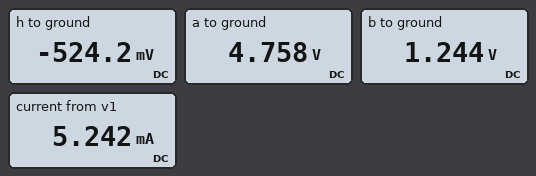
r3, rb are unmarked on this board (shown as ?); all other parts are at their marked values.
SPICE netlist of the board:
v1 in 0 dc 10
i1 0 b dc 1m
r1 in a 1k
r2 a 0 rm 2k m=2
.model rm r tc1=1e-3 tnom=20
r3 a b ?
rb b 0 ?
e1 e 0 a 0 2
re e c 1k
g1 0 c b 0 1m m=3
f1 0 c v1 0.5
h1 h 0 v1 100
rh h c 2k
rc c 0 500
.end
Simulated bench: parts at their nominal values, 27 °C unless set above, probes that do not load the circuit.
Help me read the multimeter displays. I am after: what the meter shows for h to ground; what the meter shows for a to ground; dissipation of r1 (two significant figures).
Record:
-524.2 mV
4.758 V
27 mW
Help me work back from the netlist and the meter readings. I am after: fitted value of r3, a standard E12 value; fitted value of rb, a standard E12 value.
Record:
6.8 kΩ
820 Ω
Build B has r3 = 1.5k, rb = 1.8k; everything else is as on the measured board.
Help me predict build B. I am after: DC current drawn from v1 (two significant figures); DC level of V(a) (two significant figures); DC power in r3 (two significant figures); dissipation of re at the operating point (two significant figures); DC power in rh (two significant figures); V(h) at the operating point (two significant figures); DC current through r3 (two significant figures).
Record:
5.4 mA
4.6 V
1.1 mW
21 mW
13 mW
-540 mV
850 µA
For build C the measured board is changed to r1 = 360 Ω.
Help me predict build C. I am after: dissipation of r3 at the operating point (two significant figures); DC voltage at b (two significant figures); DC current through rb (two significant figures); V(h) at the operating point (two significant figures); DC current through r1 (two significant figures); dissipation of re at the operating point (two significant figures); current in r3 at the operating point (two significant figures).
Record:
4.7 mW
1.5 V
1.8 mA
-790 mV
7.9 mA
100 mW
830 µA
